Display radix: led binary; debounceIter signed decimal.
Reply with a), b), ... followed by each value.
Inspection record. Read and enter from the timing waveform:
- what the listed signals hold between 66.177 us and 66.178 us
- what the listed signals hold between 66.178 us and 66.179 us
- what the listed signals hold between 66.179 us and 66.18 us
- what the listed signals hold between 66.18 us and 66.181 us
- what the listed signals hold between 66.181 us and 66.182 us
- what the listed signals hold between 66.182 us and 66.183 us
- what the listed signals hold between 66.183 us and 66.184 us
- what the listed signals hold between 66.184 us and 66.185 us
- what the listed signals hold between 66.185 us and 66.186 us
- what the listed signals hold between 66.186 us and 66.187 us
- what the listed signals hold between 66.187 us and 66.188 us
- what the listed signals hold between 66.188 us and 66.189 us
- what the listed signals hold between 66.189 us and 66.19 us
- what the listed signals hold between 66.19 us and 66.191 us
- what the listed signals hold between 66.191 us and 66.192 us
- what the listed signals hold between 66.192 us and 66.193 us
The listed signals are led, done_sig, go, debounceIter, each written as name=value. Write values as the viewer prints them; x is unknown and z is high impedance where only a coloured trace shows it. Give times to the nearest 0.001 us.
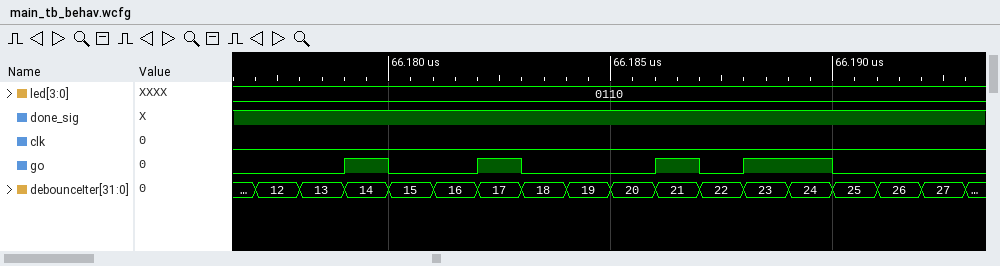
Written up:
a) led=0110, done_sig=1, go=0, debounceIter=12
b) led=0110, done_sig=1, go=0, debounceIter=13
c) led=0110, done_sig=1, go=1, debounceIter=14
d) led=0110, done_sig=1, go=0, debounceIter=15
e) led=0110, done_sig=1, go=0, debounceIter=16
f) led=0110, done_sig=1, go=1, debounceIter=17
g) led=0110, done_sig=1, go=0, debounceIter=18
h) led=0110, done_sig=1, go=0, debounceIter=19
i) led=0110, done_sig=1, go=0, debounceIter=20
j) led=0110, done_sig=1, go=1, debounceIter=21
k) led=0110, done_sig=1, go=0, debounceIter=22
l) led=0110, done_sig=1, go=1, debounceIter=23
m) led=0110, done_sig=1, go=1, debounceIter=24
n) led=0110, done_sig=1, go=0, debounceIter=25
o) led=0110, done_sig=1, go=0, debounceIter=26
p) led=0110, done_sig=1, go=0, debounceIter=27
